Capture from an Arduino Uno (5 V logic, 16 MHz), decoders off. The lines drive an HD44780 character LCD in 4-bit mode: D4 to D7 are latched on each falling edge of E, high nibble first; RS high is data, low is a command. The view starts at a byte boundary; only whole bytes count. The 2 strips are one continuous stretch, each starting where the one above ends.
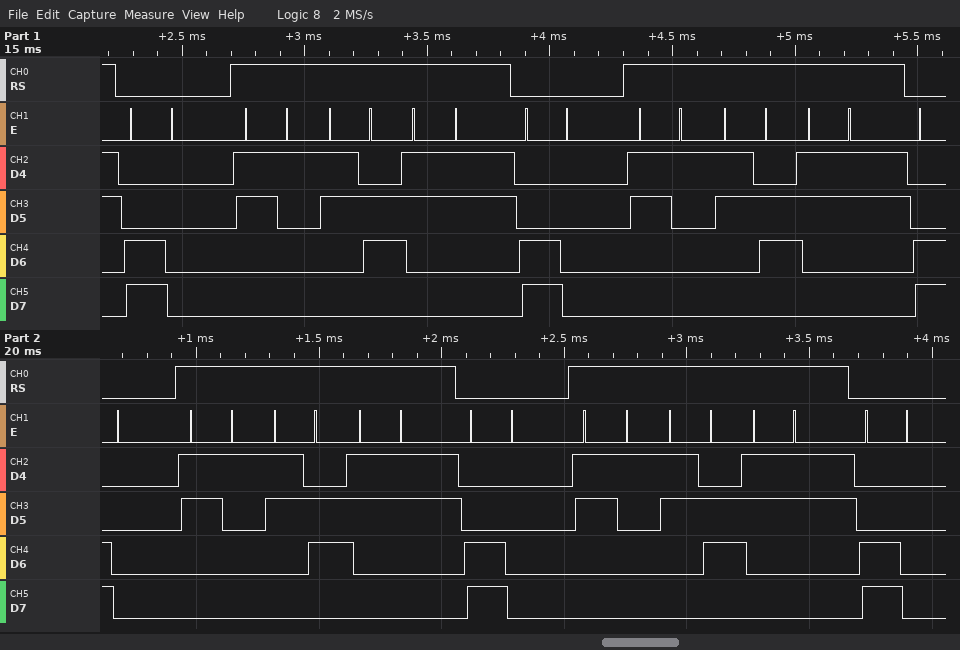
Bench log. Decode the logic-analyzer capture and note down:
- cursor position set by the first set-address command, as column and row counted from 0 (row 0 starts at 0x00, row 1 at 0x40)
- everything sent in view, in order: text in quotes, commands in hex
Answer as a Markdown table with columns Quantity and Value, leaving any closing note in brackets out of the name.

| Quantity | Value |
|---|---|
| cursor position set by the first set-address command, as column and row counted from 0 | column 0, row 1 |
| everything sent in view, in order: text in quotes, commands in hex | 0xC0 "163" 0xC0 "163" 0xC0 "163" 0xC0 "163" 0xC0 |
